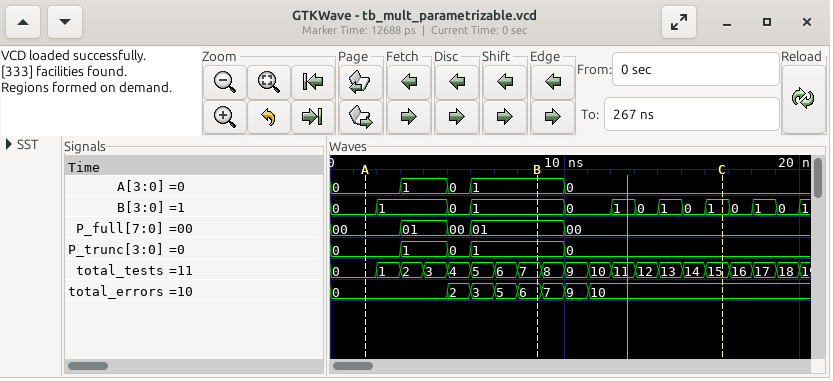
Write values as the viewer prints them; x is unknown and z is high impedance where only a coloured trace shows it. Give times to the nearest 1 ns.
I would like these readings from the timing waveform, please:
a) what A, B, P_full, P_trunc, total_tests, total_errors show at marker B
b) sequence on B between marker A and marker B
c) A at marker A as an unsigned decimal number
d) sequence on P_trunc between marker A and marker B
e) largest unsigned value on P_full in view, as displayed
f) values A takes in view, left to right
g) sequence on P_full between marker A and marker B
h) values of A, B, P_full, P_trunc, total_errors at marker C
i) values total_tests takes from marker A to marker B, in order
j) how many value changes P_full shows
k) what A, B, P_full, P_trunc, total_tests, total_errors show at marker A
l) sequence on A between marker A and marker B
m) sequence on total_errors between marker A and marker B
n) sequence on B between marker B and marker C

A=1, B=1, P_full=01, P_trunc=1, total_tests=7, total_errors=6
0, 1, 0, 1
0
0, 1, 0, 1
01
0, 1, 0, 1, 0
00, 01, 00, 01
A=0, B=1, P_full=00, P_trunc=0, total_errors=10
0, 1, 2, 3, 4, 5, 6, 7
4
A=0, B=0, P_full=00, P_trunc=0, total_tests=0, total_errors=0
0, 1, 0, 1
0, 2, 3, 5, 6
1, 0, 1, 0, 1, 0, 1
